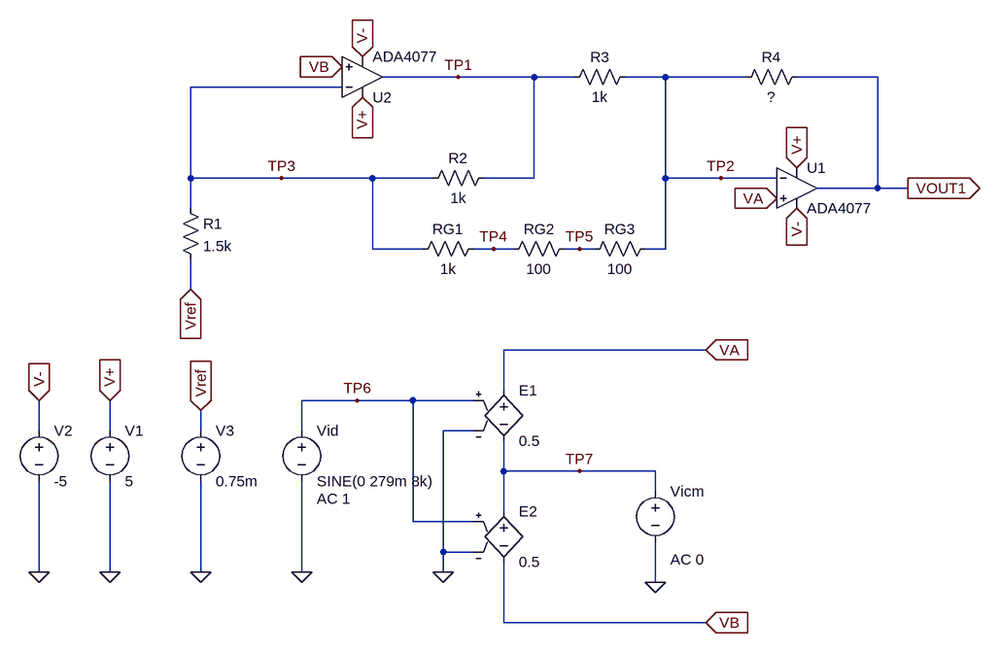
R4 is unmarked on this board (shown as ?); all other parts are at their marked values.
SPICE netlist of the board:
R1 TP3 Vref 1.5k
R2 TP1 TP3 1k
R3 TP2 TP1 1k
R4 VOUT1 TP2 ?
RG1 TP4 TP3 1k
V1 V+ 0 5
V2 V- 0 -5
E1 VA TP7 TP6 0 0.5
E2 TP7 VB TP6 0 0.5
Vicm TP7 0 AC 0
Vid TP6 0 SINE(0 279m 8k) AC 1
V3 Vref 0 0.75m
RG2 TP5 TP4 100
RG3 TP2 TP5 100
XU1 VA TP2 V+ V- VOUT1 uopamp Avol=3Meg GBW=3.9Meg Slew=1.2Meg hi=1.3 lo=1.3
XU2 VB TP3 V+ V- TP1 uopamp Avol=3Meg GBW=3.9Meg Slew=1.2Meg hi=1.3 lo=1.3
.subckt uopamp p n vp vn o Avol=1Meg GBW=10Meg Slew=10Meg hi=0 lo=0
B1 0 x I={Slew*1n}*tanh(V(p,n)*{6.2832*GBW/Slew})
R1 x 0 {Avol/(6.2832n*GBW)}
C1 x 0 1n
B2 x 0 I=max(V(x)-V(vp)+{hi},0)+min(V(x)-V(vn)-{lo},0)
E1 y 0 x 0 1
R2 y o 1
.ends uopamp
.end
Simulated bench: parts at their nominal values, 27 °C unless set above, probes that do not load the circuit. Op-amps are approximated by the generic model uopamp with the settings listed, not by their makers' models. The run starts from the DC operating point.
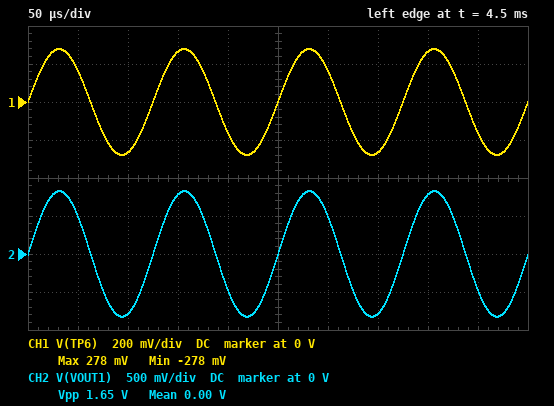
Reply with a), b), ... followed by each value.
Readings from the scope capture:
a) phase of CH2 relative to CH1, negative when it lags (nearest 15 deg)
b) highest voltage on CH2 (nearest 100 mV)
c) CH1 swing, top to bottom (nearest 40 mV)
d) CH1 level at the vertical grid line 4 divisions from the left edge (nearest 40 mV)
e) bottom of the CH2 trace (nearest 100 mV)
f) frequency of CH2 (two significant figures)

a) 0 deg
b) 800 mV
c) 560 mV
d) -160 mV
e) -800 mV
f) 8.0 kHz
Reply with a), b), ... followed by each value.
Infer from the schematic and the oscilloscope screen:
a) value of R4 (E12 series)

a) 820 Ω
